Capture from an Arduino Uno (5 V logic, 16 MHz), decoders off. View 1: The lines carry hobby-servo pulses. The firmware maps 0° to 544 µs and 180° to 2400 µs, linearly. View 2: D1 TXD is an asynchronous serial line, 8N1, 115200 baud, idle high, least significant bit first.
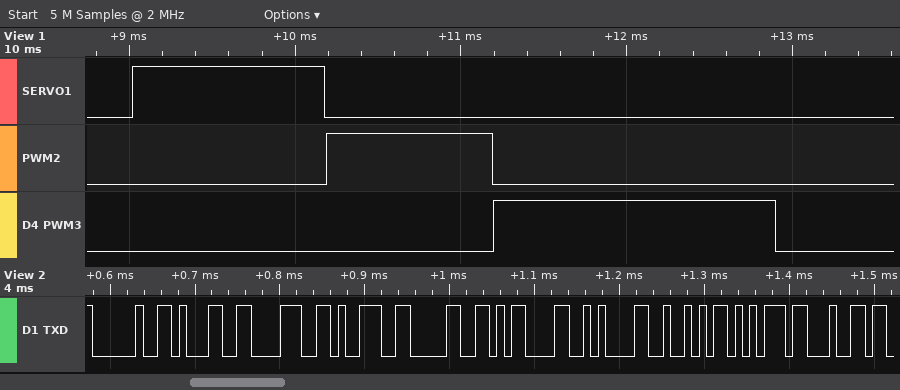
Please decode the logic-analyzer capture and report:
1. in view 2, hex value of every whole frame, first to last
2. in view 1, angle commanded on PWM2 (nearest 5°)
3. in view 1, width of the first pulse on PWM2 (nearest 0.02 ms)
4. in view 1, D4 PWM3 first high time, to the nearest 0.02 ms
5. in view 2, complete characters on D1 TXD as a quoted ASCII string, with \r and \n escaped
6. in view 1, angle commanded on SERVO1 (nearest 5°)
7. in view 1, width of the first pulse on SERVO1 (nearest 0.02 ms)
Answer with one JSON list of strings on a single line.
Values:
["20 31 38 39 30 0D 0A 52 75 64", "45°", "1.00 ms", "1.70 ms", "\" 1890\\r\\nRud\"", "60°", "1.16 ms"]
